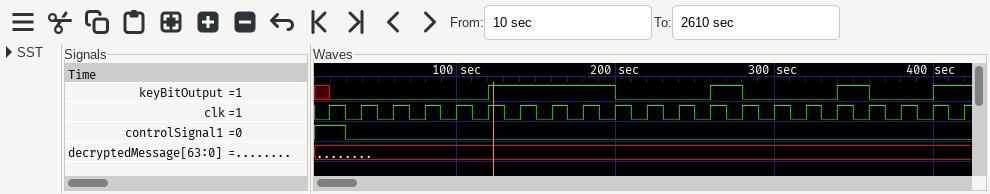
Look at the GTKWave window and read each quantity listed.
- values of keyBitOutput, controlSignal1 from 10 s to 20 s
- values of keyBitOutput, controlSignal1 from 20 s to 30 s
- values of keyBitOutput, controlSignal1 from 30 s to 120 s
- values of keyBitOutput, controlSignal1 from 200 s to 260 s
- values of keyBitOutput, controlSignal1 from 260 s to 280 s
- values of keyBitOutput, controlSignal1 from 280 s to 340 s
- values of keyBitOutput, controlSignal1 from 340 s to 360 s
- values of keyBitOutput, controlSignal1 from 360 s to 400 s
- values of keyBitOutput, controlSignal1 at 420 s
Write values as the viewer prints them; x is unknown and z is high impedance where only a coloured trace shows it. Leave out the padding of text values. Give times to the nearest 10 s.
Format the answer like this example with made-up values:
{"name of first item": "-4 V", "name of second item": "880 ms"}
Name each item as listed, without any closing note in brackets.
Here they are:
{"values of keyBitOutput, controlSignal1 from 10 s to 20 s": "keyBitOutput=x, controlSignal1=1", "values of keyBitOutput, controlSignal1 from 20 s to 30 s": "keyBitOutput=0, controlSignal1=1", "values of keyBitOutput, controlSignal1 from 30 s to 120 s": "keyBitOutput=0, controlSignal1=0", "values of keyBitOutput, controlSignal1 from 200 s to 260 s": "keyBitOutput=0, controlSignal1=0", "values of keyBitOutput, controlSignal1 from 260 s to 280 s": "keyBitOutput=1, controlSignal1=0", "values of keyBitOutput, controlSignal1 from 280 s to 340 s": "keyBitOutput=0, controlSignal1=0", "values of keyBitOutput, controlSignal1 from 340 s to 360 s": "keyBitOutput=1, controlSignal1=0", "values of keyBitOutput, controlSignal1 from 360 s to 400 s": "keyBitOutput=0, controlSignal1=0", "values of keyBitOutput, controlSignal1 at 420 s": "keyBitOutput=1, controlSignal1=0"}
